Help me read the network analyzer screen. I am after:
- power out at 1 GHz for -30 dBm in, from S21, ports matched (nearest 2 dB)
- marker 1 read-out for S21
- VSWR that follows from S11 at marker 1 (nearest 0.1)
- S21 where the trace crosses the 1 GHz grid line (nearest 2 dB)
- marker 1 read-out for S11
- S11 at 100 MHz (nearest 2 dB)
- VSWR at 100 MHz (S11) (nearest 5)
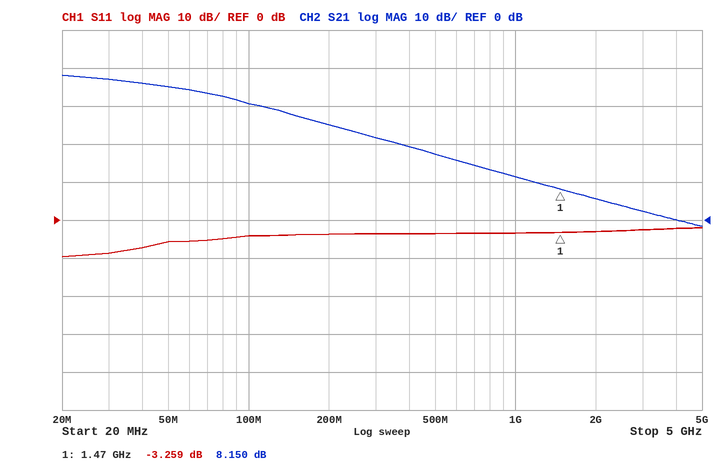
-18 dBm
8.150 dB
5.4
12 dB
-3.259 dB
-4 dB
5
